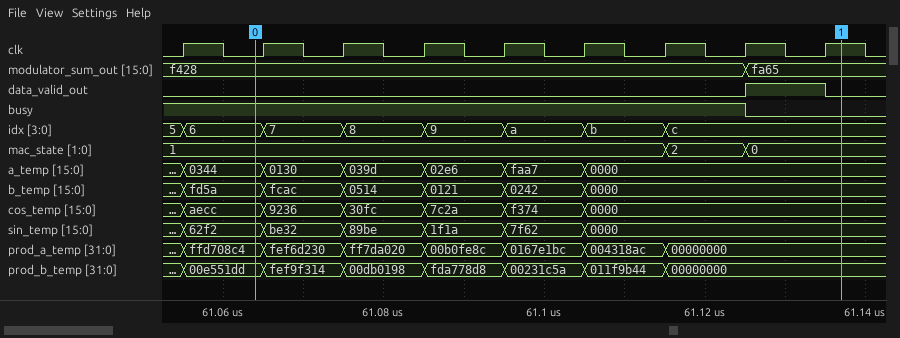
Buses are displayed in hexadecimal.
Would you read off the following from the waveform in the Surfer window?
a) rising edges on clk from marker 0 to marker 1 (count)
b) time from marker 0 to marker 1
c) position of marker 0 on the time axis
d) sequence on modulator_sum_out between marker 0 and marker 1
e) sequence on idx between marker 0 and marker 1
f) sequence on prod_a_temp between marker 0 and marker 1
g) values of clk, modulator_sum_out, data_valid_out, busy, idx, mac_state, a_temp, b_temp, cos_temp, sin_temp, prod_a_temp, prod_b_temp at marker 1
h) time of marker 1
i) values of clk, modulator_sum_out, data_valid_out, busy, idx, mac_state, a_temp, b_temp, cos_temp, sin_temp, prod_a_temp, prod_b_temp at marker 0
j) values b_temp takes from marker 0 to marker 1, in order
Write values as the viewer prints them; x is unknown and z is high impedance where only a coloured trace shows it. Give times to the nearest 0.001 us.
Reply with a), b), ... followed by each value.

a) 8
b) 0.073 us
c) 61.064 us
d) f428, fa65
e) 6, 7, 8, 9, a, b, c
f) ffd708c4, fef6d230, ff7da020, 00b0fe8c, 0167e1bc, 004318ac, 00000000
g) clk=1, modulator_sum_out=fa65, data_valid_out=0, busy=0, idx=c, mac_state=0, a_temp=0000, b_temp=0000, cos_temp=0000, sin_temp=0000, prod_a_temp=00000000, prod_b_temp=00000000
h) 61.137 us
i) clk=0, modulator_sum_out=f428, data_valid_out=0, busy=1, idx=6, mac_state=1, a_temp=0344, b_temp=fd5a, cos_temp=aecc, sin_temp=62f2, prod_a_temp=ffd708c4, prod_b_temp=00e551dd
j) fd5a, fcac, 0514, 0121, 0242, 0000
